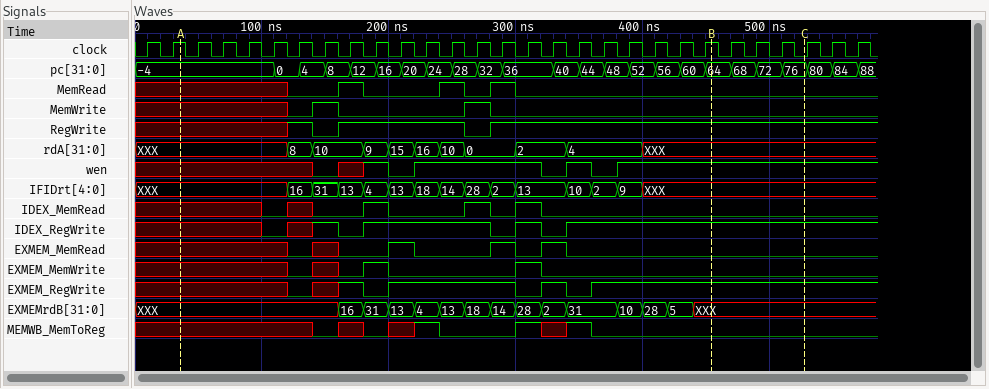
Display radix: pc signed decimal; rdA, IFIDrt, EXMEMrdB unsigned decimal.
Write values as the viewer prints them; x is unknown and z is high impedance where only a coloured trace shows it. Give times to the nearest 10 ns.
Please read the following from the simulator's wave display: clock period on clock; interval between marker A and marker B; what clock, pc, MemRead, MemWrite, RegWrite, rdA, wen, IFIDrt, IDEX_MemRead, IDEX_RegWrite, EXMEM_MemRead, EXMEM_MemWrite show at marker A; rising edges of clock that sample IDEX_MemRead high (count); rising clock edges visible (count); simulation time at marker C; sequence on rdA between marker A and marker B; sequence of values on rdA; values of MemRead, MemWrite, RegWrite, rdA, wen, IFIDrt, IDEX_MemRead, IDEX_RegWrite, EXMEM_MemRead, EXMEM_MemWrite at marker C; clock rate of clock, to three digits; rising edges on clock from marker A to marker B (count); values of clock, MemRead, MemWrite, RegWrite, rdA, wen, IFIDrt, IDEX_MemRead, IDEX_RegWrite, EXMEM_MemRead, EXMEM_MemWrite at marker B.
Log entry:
20 ns
420 ns
clock=1, pc=-4, MemRead=x, MemWrite=x, RegWrite=x, rdA=XXX, wen=x, IFIDrt=XXX, IDEX_MemRead=x, IDEX_RegWrite=x, EXMEM_MemRead=x, EXMEM_MemWrite=x
3
29
530 ns
XXX, 8, 10, 9, 15, 16, 10, 0, 2, 4, XXX
XXX, 8, 10, 9, 15, 16, 10, 0, 2, 4, XXX
MemRead=0, MemWrite=0, RegWrite=1, rdA=XXX, wen=1, IFIDrt=XXX, IDEX_MemRead=0, IDEX_RegWrite=1, EXMEM_MemRead=0, EXMEM_MemWrite=0
50.0 MHz
21
clock=1, MemRead=0, MemWrite=0, RegWrite=1, rdA=XXX, wen=1, IFIDrt=XXX, IDEX_MemRead=0, IDEX_RegWrite=1, EXMEM_MemRead=0, EXMEM_MemWrite=0
